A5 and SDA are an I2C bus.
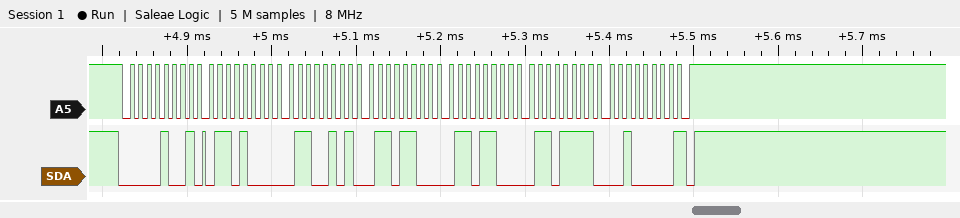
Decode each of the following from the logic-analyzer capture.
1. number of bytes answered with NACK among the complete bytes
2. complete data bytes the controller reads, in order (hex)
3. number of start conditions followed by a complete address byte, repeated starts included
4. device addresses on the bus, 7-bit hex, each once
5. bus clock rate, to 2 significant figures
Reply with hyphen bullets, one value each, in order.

- 1
- 68 65 6C 6C 6F 20
- 1
- 0x04
- 100 kHz
